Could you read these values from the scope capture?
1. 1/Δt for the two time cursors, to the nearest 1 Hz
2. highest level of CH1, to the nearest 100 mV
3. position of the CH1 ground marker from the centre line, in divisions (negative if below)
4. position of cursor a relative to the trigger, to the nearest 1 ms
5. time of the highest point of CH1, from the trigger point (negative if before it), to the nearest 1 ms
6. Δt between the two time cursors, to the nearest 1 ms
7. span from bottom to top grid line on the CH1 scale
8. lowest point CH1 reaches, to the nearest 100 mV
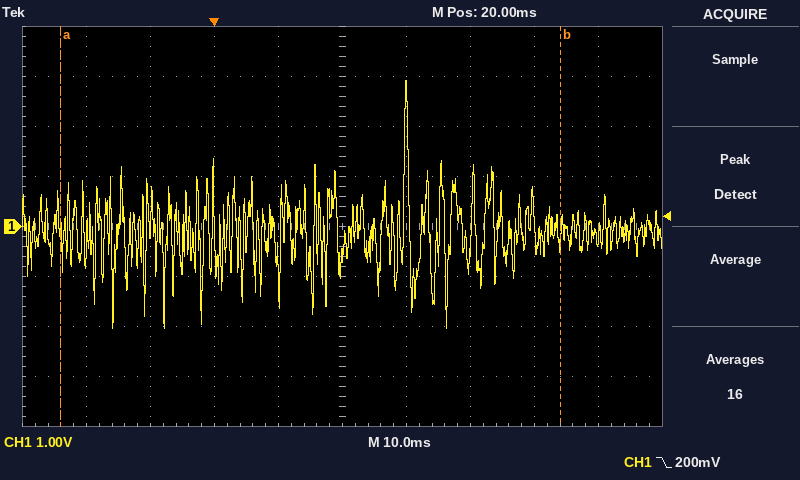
13 Hz
2.9 V
0.0 div
-24 ms
+30 ms
78 ms
8 V
-2.0 V
